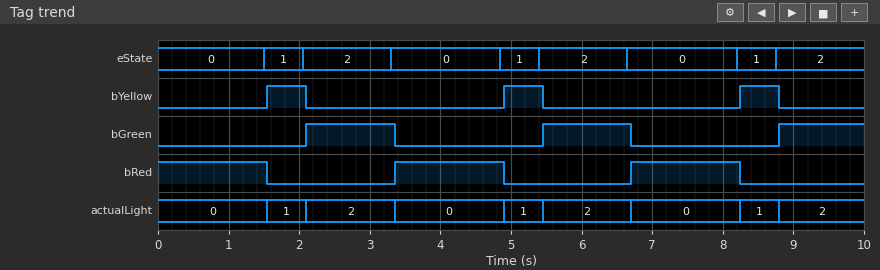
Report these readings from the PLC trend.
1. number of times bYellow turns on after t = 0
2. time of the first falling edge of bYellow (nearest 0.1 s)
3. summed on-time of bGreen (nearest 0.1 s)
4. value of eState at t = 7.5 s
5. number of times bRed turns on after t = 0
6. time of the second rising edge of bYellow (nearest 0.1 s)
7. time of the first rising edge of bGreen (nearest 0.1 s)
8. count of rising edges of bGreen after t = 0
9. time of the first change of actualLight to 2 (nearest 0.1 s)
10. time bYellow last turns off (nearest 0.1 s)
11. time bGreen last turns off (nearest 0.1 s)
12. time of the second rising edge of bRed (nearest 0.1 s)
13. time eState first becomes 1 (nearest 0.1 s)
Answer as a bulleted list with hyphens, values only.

- 3
- 2.1 s
- 3.7 s
- 0
- 2
- 4.9 s
- 2.1 s
- 3
- 2.1 s
- 8.8 s
- 6.7 s
- 6.7 s
- 1.5 s
